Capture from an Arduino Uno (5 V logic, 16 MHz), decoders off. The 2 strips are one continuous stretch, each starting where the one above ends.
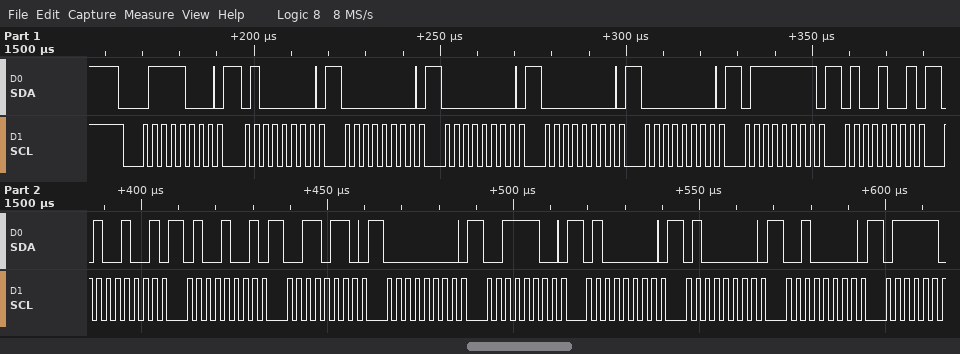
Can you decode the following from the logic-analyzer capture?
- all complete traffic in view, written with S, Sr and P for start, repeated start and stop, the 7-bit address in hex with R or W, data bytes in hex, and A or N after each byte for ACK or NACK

S 3CW A 40 A 00 A 00 A 00 A 00 A 7F A 49 A 49 A 49 A 36 A 00 A 3C A 40 A 40 A 20 A
